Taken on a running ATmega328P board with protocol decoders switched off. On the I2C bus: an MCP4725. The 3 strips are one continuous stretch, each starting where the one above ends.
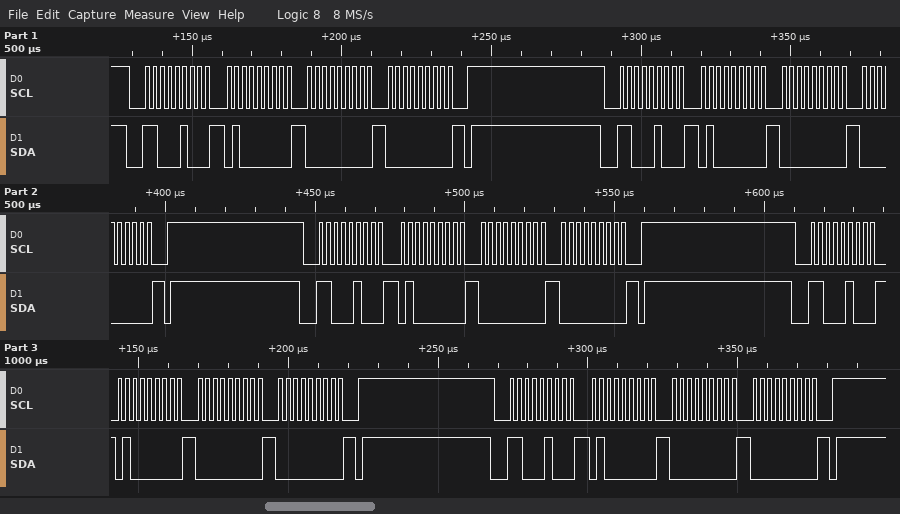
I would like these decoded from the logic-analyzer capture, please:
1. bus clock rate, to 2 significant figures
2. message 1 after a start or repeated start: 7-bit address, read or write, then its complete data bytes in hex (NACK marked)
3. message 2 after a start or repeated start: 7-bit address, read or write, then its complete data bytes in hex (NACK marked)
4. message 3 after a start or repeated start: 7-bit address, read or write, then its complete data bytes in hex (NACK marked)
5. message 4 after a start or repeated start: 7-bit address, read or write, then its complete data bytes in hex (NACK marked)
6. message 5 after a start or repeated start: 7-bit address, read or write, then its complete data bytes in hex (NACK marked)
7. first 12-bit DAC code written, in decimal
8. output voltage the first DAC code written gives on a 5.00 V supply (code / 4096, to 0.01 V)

400 kHz
0x62 write: 40 00 00
0x62 write: 40 00 00
0x62 write: 40 00 00
0x62 write: 40 00 00
0x62 write: 40 00 00
0
0.00 V
